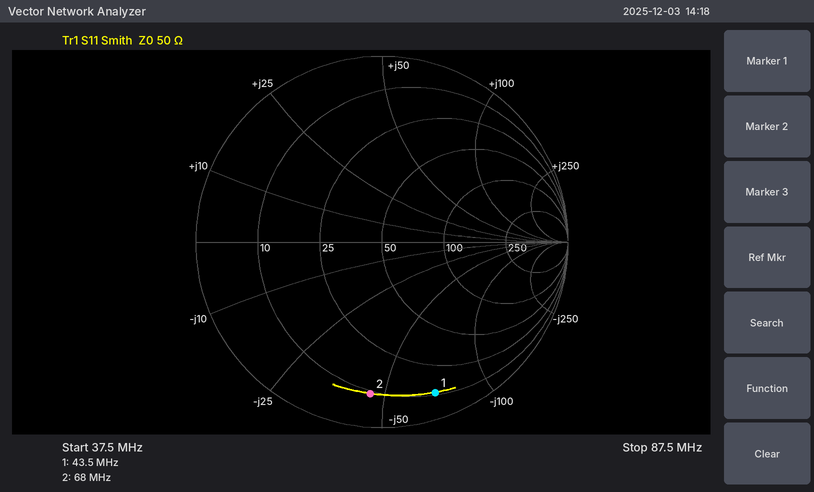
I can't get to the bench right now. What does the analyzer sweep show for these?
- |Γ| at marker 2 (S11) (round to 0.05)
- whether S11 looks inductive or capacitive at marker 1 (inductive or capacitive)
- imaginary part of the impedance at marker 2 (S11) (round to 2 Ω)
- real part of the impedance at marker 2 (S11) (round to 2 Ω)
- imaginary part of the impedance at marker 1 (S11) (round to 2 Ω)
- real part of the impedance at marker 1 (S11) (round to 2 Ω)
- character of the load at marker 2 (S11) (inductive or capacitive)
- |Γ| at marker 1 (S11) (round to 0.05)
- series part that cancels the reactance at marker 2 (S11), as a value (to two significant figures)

0.80
capacitive
-46 Ω
10 Ω
-70 Ω
12 Ω
capacitive
0.85
110 nH
